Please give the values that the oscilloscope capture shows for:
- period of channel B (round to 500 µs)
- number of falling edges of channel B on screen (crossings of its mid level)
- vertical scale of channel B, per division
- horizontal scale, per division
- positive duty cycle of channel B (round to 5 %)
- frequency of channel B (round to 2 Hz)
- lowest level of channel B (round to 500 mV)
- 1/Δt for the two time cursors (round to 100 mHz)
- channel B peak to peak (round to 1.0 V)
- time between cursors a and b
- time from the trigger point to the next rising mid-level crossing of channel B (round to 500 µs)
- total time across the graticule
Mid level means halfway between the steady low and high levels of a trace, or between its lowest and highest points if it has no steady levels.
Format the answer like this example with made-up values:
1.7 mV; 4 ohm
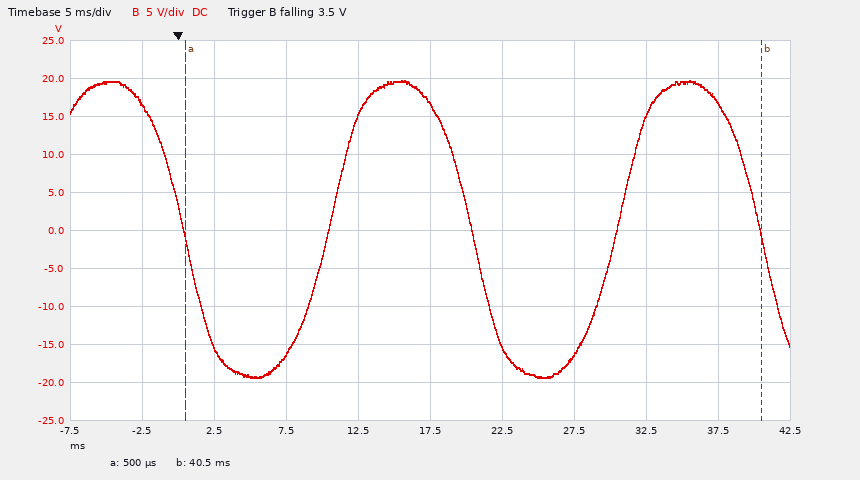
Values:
20.0 ms; 3; 5 V; 5 ms; 50 %; 50 Hz; -19.5 V; 25.0 Hz; 39.0 V; 40.0 ms; 10.5 ms; 50 ms
